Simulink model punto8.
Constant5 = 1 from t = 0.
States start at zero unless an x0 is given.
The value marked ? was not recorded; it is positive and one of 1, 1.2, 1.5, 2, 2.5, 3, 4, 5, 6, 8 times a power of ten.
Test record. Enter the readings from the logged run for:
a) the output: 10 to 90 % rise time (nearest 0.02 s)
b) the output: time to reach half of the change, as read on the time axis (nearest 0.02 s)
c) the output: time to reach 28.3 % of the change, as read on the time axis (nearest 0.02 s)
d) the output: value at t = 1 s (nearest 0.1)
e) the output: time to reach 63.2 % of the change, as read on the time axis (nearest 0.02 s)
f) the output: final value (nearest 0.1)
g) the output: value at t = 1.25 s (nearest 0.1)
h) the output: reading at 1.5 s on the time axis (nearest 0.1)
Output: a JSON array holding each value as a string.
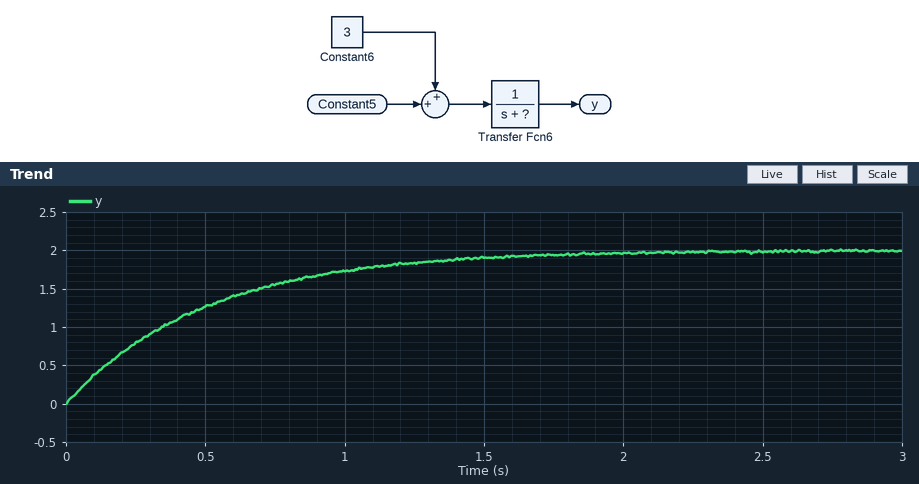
["1.10 s", "0.34 s", "0.16 s", "1.7", "0.50 s", "2.0", "1.8", "1.9"]
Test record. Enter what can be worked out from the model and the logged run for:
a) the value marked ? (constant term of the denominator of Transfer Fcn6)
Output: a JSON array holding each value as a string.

["2"]
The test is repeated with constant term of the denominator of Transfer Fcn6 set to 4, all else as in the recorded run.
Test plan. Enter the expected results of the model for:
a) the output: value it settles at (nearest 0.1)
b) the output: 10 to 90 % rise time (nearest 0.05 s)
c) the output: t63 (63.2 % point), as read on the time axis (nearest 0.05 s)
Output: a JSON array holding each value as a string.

["1.0", "0.55 s", "0.25 s"]
